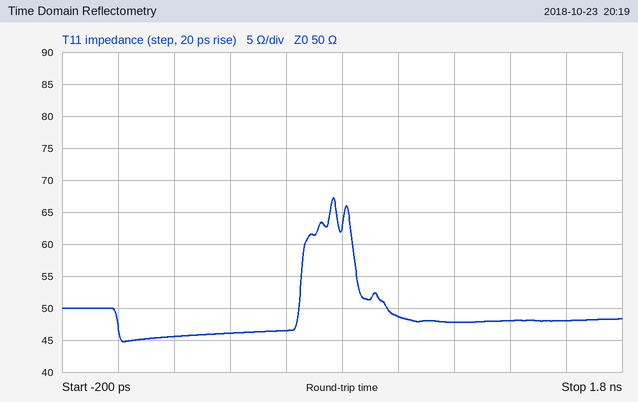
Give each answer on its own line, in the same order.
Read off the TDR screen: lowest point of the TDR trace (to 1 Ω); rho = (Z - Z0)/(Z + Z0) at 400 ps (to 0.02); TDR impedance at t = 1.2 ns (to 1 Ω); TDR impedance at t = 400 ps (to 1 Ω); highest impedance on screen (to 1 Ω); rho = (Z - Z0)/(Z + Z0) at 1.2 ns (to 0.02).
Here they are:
45 Ω
-0.04
48 Ω
46 Ω
67 Ω
-0.02
